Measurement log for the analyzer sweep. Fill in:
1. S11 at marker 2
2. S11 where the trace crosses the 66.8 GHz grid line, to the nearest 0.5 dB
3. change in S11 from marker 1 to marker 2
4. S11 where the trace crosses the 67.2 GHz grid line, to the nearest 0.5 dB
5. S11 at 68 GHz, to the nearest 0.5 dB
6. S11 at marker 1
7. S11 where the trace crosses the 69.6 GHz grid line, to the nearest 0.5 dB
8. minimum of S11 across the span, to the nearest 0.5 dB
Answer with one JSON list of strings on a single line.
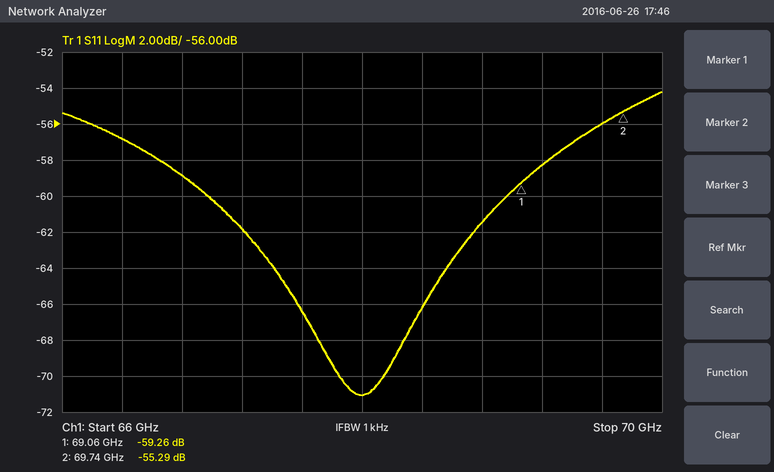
["-55.29 dB", "-59.0 dB", "3.97 dB", "-62.0 dB", "-71.0 dB", "-59.26 dB", "-56.0 dB", "-71.0 dB"]
